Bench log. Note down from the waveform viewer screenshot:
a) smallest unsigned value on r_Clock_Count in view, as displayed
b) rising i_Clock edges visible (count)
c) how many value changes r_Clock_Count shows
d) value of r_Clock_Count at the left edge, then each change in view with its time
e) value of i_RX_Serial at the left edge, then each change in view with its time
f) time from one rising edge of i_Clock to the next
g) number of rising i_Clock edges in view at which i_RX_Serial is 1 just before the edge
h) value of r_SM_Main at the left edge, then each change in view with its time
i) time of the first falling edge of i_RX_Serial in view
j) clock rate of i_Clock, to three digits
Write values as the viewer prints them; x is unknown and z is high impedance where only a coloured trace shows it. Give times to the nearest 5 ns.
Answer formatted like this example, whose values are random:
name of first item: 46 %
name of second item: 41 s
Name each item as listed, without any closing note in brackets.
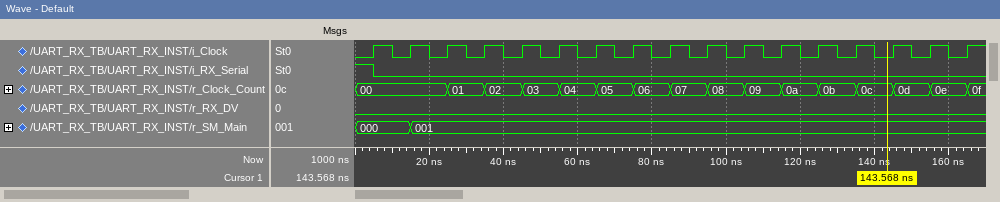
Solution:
smallest unsigned value on r_Clock_Count in view, as displayed: 00
rising i_Clock edges visible: 17
how many value changes r_Clock_Count shows: 15
value of r_Clock_Count at the left edge, then each change in view with its time: 00, 01 at 25 ns, 02 at 35 ns, 03 at 45 ns, 04 at 55 ns, 05 at 65 ns, 06 at 75 ns, 07 at 85 ns, 08 at 95 ns, 09 at 105 ns, 0a at 115 ns, 0b at 125 ns, 0c at 135 ns, 0d at 145 ns, 0e at 155 ns, 0f at 165 ns
value of i_RX_Serial at the left edge, then each change in view with its time: 1, 0 at 5 ns
time from one rising edge of i_Clock to the next: 10 ns
number of rising i_Clock edges in view at which i_RX_Serial is 1 just before the edge: 1
value of r_SM_Main at the left edge, then each change in view with its time: 000, 001 at 15 ns
time of the first falling edge of i_RX_Serial in view: 5 ns
clock rate of i_Clock, to three digits: 100 MHz
